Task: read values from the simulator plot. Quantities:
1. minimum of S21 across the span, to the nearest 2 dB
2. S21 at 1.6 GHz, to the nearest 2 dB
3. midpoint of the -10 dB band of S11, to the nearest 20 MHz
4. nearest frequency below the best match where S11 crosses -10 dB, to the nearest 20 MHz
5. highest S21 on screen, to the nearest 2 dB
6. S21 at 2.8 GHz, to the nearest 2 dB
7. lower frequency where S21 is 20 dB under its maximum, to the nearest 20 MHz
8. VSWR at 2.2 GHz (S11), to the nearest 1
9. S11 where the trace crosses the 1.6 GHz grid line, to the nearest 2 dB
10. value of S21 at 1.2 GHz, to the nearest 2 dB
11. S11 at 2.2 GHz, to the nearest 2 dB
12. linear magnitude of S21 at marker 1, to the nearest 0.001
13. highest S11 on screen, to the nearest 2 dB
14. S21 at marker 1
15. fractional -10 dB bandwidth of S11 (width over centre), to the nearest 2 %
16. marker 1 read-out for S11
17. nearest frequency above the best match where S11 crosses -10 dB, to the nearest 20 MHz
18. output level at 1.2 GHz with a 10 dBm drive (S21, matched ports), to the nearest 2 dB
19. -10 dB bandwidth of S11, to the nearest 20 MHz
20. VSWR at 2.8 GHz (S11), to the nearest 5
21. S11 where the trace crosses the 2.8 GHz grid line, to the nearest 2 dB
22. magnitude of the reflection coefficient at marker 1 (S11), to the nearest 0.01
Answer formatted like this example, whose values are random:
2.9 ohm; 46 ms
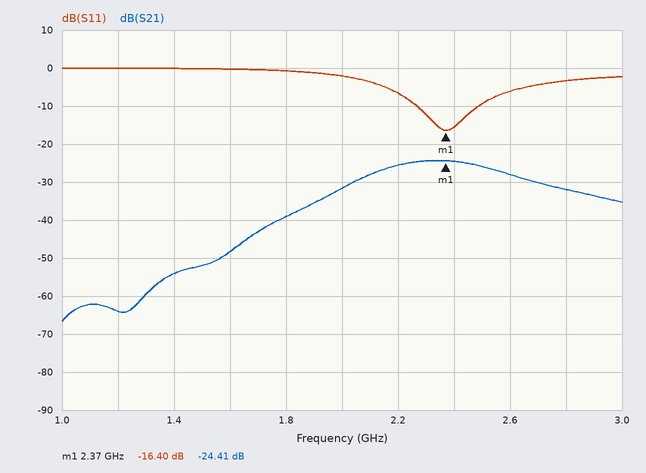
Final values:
-66 dB; -48 dB; 2.38 GHz; 2.26 GHz; -24 dB; -32 dB; 1.68 GHz; 3; 0 dB; -64 dB; -6 dB; 0.060; 0 dB; -24.41 dB; 10 %; -16.40 dB; 2.48 GHz; -54 dBm; 220 MHz; 5; -4 dB; 0.15
